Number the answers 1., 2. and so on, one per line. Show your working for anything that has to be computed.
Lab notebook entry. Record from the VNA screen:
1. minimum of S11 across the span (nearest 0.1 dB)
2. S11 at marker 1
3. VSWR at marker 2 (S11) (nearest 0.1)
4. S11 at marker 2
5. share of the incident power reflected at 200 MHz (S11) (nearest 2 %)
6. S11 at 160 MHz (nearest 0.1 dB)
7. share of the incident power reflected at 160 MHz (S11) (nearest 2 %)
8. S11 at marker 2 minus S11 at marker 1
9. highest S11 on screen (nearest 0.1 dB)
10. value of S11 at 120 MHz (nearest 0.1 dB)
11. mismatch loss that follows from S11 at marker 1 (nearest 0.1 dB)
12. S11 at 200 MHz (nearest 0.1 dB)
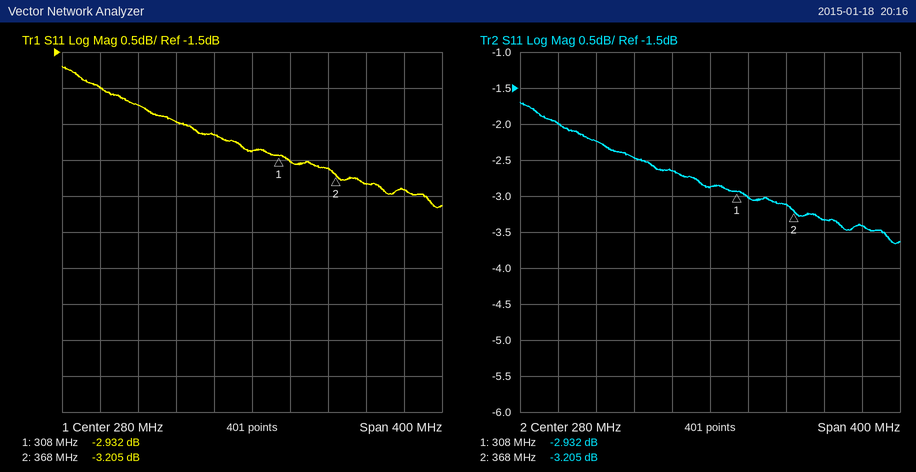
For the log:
1. -3.7 dB
2. -2.932 dB
3. (1 + 0.6914)/(1 − 0.6914) ≈ 5.5
4. -3.205 dB
5. 10^(-2.5/10) ≈ 56 %
6. -2.2 dB
7. 10^(-2.2/10) ≈ 60 %
8. -3.205 − (-2.932) = -0.273 dB
9. -1.7 dB
10. -2.0 dB
11. −10 log10(1 − 10^(-2.932/10)) ≈ 3.1 dB
12. -2.5 dB
